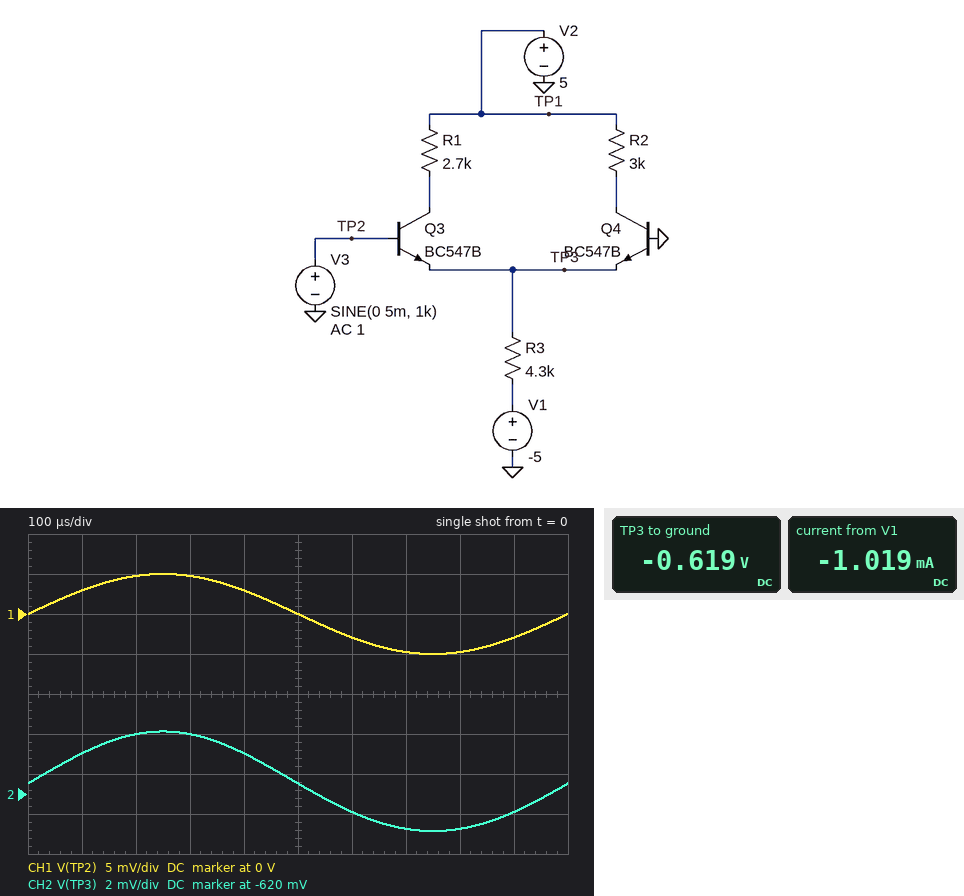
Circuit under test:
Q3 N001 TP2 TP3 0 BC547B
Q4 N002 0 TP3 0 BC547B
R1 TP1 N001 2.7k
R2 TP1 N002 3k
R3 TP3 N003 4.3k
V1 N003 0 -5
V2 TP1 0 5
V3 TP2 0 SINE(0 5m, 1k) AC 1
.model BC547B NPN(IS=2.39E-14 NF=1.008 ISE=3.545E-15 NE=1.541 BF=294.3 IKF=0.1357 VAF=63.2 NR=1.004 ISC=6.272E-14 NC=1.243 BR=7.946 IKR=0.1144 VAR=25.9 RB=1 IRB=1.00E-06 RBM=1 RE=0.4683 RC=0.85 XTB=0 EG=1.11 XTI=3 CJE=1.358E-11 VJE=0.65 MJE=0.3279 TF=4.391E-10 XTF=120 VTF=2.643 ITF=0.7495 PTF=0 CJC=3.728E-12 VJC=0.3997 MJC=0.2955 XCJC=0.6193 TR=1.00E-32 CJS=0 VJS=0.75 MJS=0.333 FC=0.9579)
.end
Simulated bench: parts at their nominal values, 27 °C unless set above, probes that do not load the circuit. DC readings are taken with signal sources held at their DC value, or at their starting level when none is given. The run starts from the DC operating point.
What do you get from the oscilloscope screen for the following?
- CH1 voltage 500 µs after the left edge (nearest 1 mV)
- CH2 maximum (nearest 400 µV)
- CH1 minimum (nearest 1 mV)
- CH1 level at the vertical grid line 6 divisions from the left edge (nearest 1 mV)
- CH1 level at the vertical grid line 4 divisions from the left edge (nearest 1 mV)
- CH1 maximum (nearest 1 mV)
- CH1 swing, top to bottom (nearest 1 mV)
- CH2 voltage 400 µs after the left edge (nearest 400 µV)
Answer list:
0 V
-616.8 mV
-5 mV
-3 mV
3 mV
5 mV
10 mV
-618.0 mV
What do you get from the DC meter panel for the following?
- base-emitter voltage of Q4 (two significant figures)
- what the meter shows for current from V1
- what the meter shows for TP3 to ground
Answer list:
620 mV
-1.019 mA
-0.619 V
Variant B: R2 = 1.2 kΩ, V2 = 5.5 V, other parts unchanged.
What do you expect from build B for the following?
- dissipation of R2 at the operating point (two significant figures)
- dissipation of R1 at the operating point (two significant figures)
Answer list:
310 µW
690 µW
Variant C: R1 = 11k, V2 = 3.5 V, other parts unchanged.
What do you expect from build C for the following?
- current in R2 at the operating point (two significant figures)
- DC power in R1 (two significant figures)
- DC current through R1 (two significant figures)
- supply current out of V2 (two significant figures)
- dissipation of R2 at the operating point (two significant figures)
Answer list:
610 µA
1.5 mW
370 µA
980 µA
1.1 mW
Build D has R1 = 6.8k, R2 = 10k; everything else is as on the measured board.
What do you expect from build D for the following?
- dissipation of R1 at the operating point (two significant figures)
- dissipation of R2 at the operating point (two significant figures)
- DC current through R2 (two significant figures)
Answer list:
1.8 mW
2.5 mW
500 µA
